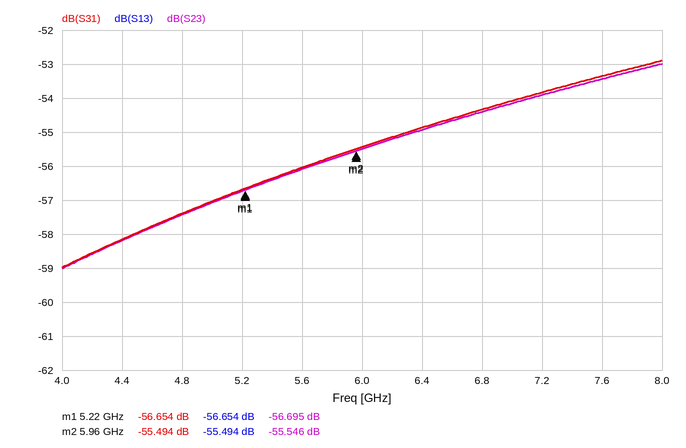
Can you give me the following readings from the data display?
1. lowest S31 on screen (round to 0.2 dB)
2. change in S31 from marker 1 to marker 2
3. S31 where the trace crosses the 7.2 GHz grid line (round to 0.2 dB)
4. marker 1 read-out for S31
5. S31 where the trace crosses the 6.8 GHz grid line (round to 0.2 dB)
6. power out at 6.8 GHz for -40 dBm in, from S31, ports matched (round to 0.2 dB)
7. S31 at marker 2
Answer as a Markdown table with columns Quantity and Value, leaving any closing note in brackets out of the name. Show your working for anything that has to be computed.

| Quantity | Value |
|---|---|
| lowest S31 on screen | -59.0 dB |
| change in S31 from marker 1 to marker 2 | -55.494 − (-56.654) = 1.160 dB |
| S31 where the trace crosses the 7.2 GHz grid line | -53.8 dB |
| marker 1 read-out for S31 | -56.654 dB |
| S31 where the trace crosses the 6.8 GHz grid line | -54.4 dB |
| power out at 6.8 GHz for -40 dBm in, from S31, ports matched | -40 dBm + (-54.4 dB) = -94.4 dBm |
| S31 at marker 2 | -55.494 dB |
